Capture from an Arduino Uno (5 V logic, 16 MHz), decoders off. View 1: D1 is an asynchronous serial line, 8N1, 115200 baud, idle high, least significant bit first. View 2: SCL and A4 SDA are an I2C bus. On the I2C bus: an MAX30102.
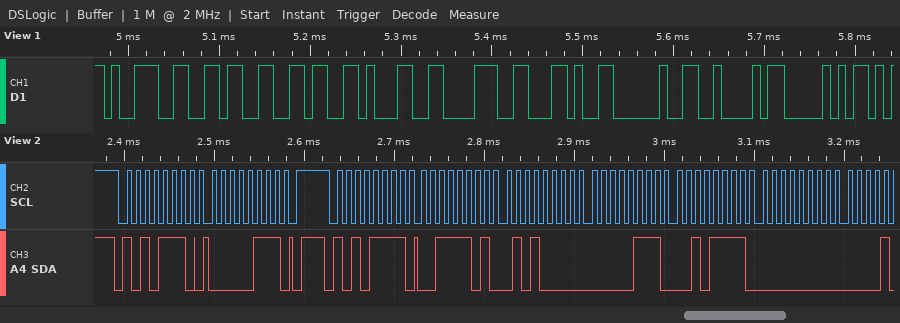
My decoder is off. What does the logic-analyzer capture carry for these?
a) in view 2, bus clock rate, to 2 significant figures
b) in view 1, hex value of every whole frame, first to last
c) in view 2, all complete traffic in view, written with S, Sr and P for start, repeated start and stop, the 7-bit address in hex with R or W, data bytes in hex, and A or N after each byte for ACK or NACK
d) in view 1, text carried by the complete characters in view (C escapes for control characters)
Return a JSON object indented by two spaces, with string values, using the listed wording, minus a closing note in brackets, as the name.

{
  "in view 2, bus clock rate, to 2 significant figures": "100 kHz",
  "in view 1, hex value of every whole frame, first to last": "39 36 36 31 38 2C 20 42 50",
  "in view 2, all complete traffic in view, written with S, Sr and P for start, repeated start and stop, the 7-bit address in hex with R or W, data bytes in hex, and A or N after each byte for ACK or NACK": "S 57W A 07 A P S 57R A 3D A 50 A 07 A 2F A 00 A",
  "in view 1, text carried by the complete characters in view": "\"96618, BP\""
}
